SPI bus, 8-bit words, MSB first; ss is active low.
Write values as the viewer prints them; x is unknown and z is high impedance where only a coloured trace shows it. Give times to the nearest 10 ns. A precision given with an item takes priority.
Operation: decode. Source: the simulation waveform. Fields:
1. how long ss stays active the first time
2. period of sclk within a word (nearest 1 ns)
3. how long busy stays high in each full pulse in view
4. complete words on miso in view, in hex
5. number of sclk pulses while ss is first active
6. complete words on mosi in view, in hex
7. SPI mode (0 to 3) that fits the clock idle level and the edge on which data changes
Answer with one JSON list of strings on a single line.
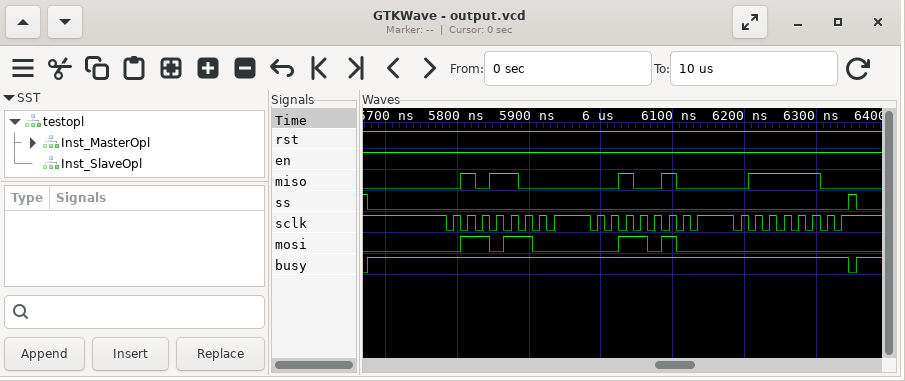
["670 ns", "20 ns", "670 ns", "58, 24, 7C", "24", "6C, 34, 00", "3"]
